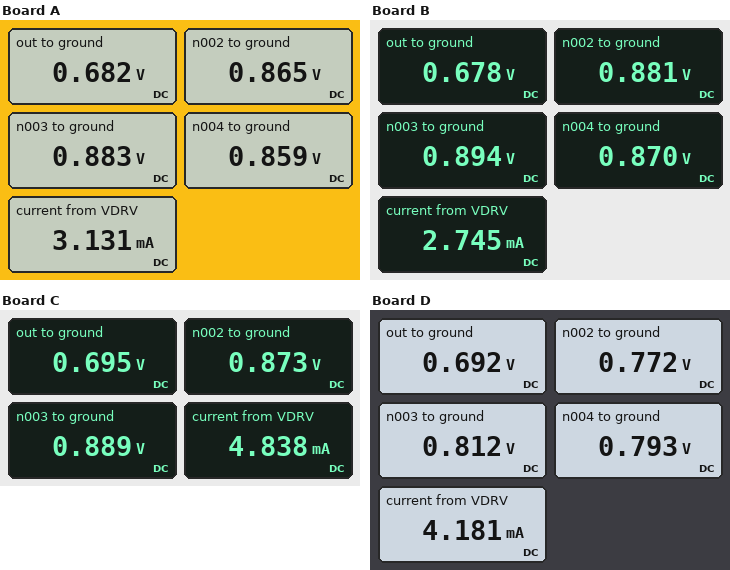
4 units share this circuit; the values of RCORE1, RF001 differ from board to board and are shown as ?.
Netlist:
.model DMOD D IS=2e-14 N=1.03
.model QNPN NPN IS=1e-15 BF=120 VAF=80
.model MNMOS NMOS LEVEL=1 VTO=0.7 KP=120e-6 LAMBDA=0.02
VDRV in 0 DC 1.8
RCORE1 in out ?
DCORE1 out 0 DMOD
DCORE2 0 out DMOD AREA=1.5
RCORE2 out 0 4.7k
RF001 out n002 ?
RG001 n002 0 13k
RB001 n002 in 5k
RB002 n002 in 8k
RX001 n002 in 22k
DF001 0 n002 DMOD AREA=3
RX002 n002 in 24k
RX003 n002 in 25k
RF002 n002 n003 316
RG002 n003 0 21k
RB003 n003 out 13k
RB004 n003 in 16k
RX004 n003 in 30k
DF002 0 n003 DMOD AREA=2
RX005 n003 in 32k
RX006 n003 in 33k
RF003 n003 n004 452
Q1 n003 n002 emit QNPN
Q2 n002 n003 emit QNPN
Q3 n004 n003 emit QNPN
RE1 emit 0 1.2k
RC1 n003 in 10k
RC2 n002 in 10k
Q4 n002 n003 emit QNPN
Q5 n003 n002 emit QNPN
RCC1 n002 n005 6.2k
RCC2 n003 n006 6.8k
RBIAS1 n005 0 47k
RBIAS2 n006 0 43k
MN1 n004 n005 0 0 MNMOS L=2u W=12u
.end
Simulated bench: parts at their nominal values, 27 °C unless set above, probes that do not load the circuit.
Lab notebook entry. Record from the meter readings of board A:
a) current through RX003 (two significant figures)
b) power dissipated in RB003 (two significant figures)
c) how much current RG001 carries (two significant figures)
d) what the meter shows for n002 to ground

37 µA
3.1 µW
67 µA
0.865 V
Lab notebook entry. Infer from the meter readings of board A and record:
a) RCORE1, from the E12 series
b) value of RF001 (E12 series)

470 Ω
470 Ω
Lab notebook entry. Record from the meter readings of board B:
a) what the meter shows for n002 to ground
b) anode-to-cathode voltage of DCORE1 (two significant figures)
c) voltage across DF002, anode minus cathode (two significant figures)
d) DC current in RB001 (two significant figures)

0.881 V
680 mV
-890 mV
180 µA
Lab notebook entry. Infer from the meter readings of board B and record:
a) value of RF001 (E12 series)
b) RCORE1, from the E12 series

560 Ω
560 Ω
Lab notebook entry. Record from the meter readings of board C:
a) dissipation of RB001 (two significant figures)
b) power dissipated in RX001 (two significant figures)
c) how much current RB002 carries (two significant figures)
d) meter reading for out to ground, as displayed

170 µW
39 µW
120 µA
0.695 V
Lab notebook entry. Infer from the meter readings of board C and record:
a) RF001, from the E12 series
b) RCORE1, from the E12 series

470 Ω
270 Ω
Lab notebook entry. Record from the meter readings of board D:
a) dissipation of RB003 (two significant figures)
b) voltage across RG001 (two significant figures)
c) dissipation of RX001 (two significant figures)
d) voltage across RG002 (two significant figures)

1.1 µW
770 mV
48 µW
810 mV
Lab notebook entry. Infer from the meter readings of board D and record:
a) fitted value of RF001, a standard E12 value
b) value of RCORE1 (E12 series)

150 Ω
330 Ω
